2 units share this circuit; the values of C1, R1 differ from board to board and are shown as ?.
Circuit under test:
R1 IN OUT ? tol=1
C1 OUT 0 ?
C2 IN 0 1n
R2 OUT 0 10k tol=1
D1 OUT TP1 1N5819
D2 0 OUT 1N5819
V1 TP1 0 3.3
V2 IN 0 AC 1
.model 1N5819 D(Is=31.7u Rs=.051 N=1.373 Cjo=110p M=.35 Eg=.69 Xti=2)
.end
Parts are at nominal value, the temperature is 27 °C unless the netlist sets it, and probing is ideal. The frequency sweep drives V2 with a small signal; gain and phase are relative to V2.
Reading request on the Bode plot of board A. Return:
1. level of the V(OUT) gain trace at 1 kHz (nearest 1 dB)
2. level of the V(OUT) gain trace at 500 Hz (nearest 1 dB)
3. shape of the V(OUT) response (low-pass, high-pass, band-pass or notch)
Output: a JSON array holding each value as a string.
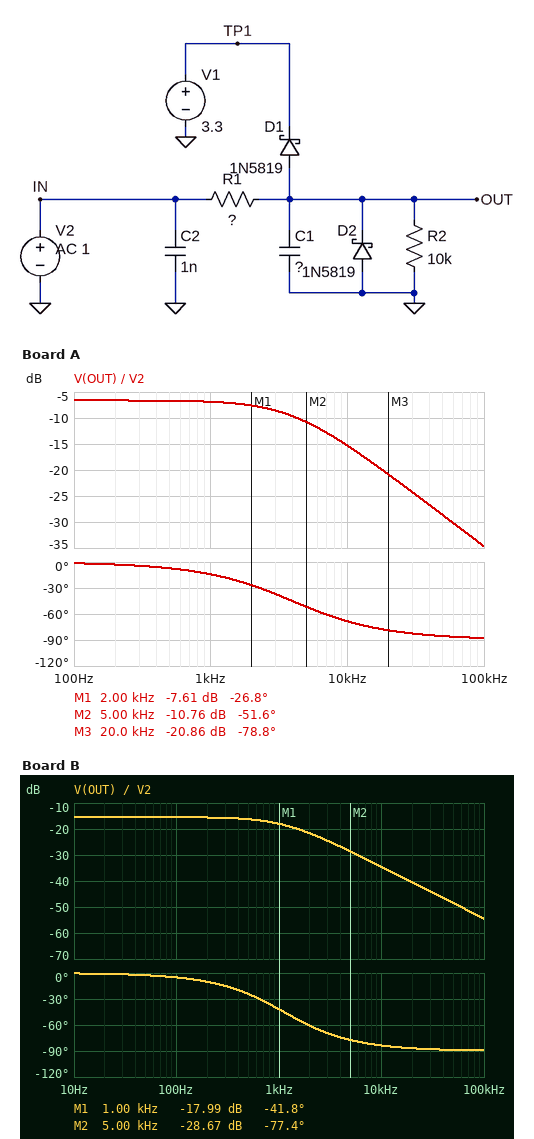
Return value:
["-7 dB", "-7 dB", "low-pass"]
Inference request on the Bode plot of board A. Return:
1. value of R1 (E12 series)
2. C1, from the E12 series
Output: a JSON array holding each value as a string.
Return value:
["2.2 kΩ", "39 nF"]
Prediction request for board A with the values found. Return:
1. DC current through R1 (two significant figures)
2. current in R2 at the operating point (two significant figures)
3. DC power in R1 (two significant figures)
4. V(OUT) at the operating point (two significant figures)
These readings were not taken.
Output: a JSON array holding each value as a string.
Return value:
["12 µA", "2.7 µA", "330 nW", "27 mV"]
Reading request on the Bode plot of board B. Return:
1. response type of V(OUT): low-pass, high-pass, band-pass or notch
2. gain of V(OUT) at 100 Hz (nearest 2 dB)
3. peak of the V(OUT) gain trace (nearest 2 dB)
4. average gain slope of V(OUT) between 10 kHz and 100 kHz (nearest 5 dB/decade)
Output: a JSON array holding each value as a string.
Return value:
["low-pass", "-16 dB", "-16 dB", "-20 dB/decade"]
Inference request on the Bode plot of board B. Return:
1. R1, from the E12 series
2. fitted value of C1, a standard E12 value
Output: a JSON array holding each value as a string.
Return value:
["15 kΩ", "56 nF"]
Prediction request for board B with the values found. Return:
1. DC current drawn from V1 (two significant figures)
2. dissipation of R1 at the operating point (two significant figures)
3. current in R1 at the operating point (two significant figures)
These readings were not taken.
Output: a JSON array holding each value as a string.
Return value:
["32 µA", "160 nW", "3.2 µA"]
